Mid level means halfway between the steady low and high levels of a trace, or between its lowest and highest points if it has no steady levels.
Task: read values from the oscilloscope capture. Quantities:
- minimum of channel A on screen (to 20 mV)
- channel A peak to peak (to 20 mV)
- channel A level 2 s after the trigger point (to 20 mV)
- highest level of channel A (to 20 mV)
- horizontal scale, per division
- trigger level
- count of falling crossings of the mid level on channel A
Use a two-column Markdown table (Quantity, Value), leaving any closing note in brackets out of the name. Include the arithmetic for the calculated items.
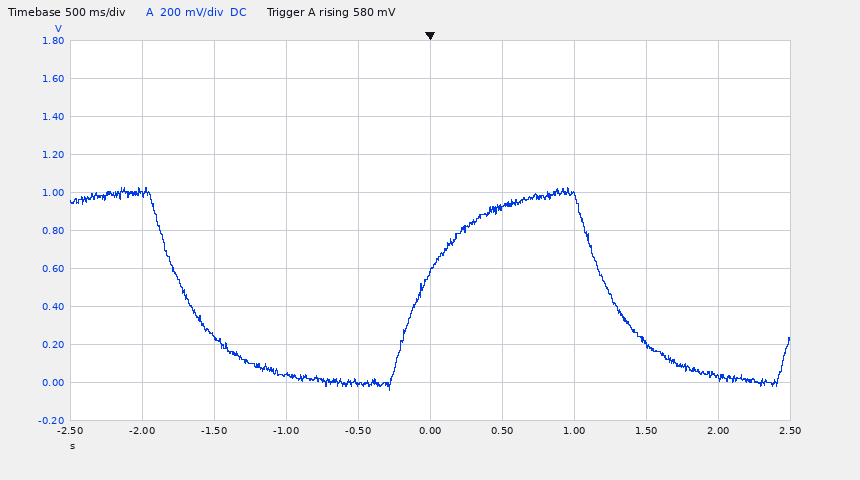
| Quantity | Value |
|---|---|
| minimum of channel A on screen | -40 mV |
| channel A peak to peak | 1.02 V − (-40 mV) = 1.06 V |
| channel A level 2 s after the trigger point | 20 mV |
| highest level of channel A | 1.02 V |
| horizontal scale, per division | 500 ms |
| trigger level | 580 mV |
| count of falling crossings of the mid level on channel A | 2 |
